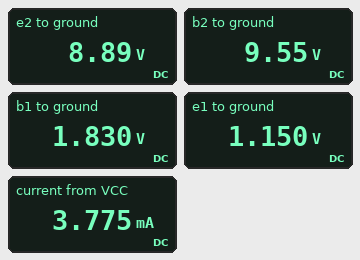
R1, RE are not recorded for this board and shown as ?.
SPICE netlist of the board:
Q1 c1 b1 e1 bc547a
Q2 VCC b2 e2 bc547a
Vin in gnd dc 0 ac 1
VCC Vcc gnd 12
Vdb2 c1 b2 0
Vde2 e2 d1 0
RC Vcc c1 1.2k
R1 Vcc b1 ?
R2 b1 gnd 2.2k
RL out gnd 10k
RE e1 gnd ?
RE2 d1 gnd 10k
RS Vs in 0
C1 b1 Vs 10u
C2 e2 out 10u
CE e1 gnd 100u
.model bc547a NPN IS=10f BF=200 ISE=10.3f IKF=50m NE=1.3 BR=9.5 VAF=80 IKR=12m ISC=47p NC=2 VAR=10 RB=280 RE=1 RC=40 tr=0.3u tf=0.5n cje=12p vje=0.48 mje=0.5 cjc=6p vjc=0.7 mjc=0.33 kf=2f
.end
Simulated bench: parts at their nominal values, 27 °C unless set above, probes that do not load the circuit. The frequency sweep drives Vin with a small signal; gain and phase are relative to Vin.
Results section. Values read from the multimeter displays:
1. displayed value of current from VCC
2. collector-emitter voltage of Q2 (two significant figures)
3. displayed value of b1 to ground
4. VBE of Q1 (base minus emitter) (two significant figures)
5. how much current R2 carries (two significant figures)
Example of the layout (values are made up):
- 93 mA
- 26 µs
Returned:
- 3.775 mA
- 3.1 V
- 1.830 V
- 680 mV
- 830 µA
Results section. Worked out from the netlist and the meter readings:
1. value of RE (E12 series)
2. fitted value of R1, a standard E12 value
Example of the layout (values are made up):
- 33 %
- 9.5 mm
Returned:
- 560 Ω
- 12 kΩ
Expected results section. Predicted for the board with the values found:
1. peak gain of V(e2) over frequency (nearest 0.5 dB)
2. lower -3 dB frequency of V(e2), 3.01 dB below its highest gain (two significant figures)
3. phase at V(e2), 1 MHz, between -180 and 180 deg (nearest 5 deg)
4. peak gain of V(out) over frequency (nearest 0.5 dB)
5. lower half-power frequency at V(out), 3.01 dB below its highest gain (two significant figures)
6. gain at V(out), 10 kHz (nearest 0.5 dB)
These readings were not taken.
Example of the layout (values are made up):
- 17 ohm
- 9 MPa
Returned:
- 37.0 dB
- 110 Hz
- 155 deg
- 37.0 dB
- 110 Hz
- 37.0 dB
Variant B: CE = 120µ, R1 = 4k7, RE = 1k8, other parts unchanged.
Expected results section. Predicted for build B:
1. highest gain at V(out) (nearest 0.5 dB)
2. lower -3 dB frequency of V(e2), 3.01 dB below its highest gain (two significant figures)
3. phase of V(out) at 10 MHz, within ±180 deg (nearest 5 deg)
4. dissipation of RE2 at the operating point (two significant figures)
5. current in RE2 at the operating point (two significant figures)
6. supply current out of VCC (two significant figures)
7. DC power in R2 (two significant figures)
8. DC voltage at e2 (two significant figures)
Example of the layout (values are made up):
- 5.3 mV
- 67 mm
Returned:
- 36.0 dB
- 79 Hz
- 90 deg
- 8.6 mW
- 930 µA
- 4.4 mA
- 6.6 mW
- 9.3 V
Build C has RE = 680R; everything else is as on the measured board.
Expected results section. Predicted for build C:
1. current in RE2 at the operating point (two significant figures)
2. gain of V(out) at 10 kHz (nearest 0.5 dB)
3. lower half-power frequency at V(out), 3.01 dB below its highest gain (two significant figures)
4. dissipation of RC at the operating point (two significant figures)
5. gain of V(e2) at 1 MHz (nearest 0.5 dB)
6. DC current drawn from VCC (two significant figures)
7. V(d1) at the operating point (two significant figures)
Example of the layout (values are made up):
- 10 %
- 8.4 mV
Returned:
- 930 µA
- 36.0 dB
- 93 Hz
- 3.5 mW
- 35.0 dB
- 3.5 mA
- 9.3 V
